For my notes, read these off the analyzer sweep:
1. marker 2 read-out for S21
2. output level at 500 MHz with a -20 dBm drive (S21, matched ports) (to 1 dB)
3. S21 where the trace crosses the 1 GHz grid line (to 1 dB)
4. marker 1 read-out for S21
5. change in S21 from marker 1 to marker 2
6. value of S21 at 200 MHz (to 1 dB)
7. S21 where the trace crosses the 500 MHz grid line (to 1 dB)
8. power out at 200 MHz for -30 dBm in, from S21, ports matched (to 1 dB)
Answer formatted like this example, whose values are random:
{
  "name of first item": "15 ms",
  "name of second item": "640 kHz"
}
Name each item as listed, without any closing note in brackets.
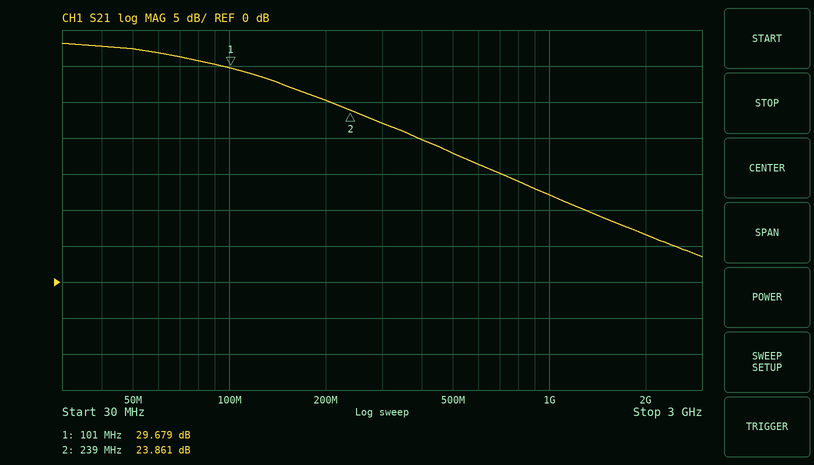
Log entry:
{
  "marker 2 read-out for S21": "23.861 dB",
  "output level at 500 MHz with a -20 dBm drive (S21, matched ports)": "-2 dBm",
  "S21 where the trace crosses the 1 GHz grid line": "12 dB",
  "marker 1 read-out for S21": "29.679 dB",
  "change in S21 from marker 1 to marker 2": "-5.818 dB",
  "value of S21 at 200 MHz": "25 dB",
  "S21 where the trace crosses the 500 MHz grid line": "18 dB",
  "power out at 200 MHz for -30 dBm in, from S21, ports matched": "-5 dBm"
}
